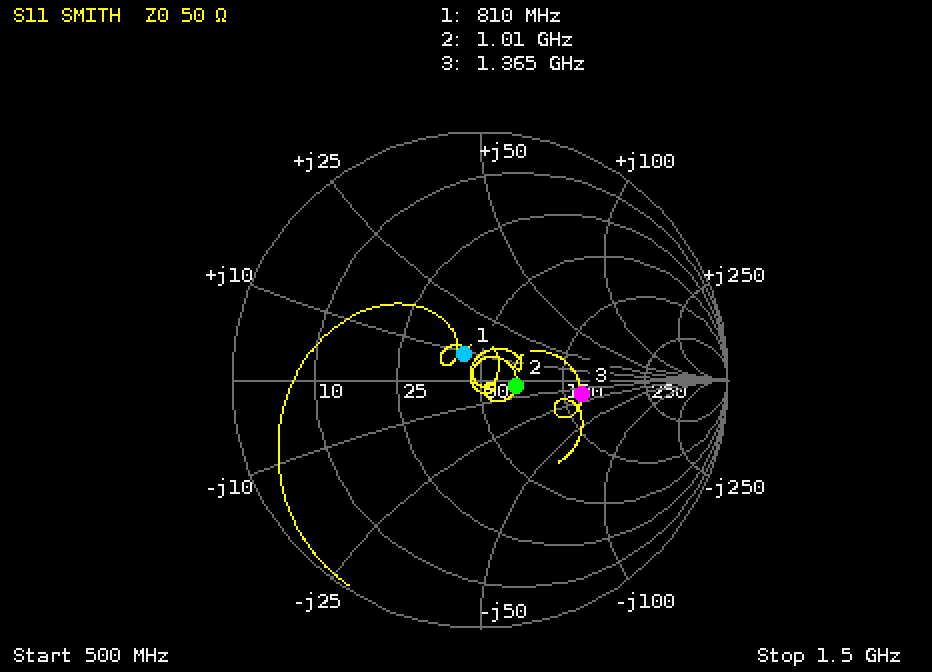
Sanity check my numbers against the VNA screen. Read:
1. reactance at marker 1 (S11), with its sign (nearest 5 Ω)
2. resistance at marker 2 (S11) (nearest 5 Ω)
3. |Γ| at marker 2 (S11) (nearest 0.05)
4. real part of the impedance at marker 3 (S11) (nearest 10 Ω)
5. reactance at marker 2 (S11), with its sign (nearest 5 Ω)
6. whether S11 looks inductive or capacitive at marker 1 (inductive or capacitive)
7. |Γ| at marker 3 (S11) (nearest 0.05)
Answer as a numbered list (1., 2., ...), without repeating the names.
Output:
1. +10 Ω
2. 65 Ω
3. 0.15
4. 120 Ω
5. -5 Ω
6. inductive
7. 0.40
